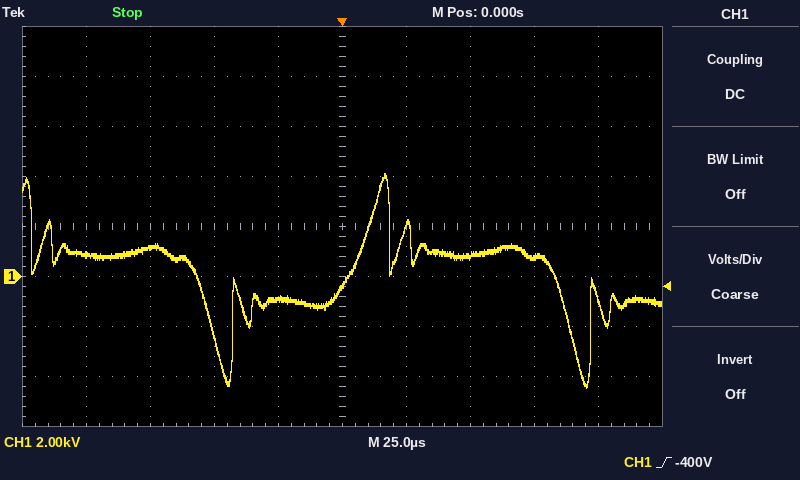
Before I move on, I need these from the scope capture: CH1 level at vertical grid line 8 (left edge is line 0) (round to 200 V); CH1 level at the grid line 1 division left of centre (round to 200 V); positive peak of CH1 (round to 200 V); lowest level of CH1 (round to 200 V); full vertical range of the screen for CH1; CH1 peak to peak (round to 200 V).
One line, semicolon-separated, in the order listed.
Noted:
800 V; -800 V; 4.2 kV; -4.4 kV; 16 kV; 8.6 kV
